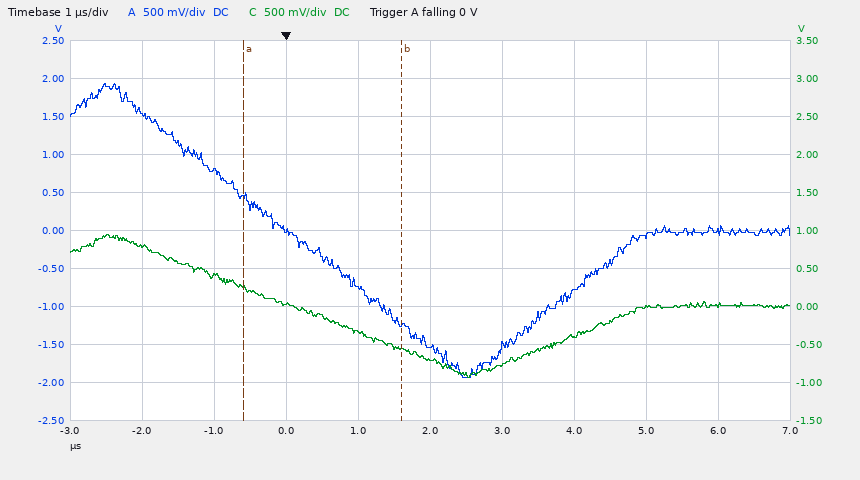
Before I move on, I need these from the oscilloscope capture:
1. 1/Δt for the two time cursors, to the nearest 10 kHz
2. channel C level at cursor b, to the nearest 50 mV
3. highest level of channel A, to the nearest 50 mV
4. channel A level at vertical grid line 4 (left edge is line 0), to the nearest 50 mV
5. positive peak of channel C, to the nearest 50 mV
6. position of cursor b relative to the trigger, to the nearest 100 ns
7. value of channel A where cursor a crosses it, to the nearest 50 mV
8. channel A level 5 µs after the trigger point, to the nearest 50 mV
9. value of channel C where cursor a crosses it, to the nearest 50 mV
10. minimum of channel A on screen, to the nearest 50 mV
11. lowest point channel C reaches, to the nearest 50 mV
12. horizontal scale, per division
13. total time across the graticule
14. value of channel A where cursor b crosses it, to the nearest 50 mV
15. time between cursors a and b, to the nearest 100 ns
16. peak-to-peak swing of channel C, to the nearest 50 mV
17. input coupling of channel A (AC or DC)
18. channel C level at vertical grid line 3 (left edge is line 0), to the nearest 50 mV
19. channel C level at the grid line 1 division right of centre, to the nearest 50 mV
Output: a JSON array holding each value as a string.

["450 kHz", "-550 mV", "1.95 V", "-750 mV", "950 mV", "+1.6 µs", "450 mV", "-50 mV", "250 mV", "-1.95 V", "-950 mV", "1 µs", "10 µs", "-1.25 V", "2.2 µs", "1.90 V", "DC", "50 mV", "-750 mV"]
